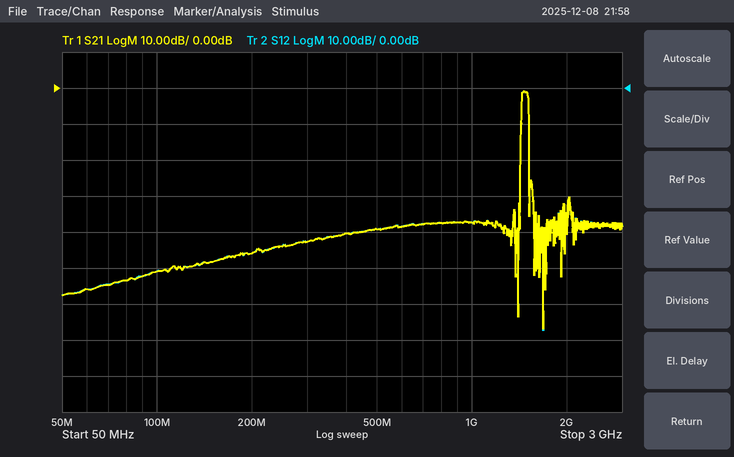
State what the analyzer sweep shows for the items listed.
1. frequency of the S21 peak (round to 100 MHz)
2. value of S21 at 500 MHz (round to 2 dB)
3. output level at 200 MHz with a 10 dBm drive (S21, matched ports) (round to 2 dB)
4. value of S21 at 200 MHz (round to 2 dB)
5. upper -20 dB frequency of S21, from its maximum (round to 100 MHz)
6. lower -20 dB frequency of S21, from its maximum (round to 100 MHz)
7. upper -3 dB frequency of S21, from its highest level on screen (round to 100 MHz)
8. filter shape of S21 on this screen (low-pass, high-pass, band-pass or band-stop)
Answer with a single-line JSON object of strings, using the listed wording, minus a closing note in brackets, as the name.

{"frequency of the S21 peak": "1.5 GHz", "value of S21 at 500 MHz": "-40 dB", "output level at 200 MHz with a 10 dBm drive (S21, matched ports)": "-36 dBm", "value of S21 at 200 MHz": "-46 dB", "upper -20 dB frequency of S21, from its maximum": "1.5 GHz", "lower -20 dB frequency of S21, from its maximum": "1.4 GHz", "upper -3 dB frequency of S21, from its highest level on screen": "1.5 GHz", "filter shape of S21 on this screen": "band-pass"}
